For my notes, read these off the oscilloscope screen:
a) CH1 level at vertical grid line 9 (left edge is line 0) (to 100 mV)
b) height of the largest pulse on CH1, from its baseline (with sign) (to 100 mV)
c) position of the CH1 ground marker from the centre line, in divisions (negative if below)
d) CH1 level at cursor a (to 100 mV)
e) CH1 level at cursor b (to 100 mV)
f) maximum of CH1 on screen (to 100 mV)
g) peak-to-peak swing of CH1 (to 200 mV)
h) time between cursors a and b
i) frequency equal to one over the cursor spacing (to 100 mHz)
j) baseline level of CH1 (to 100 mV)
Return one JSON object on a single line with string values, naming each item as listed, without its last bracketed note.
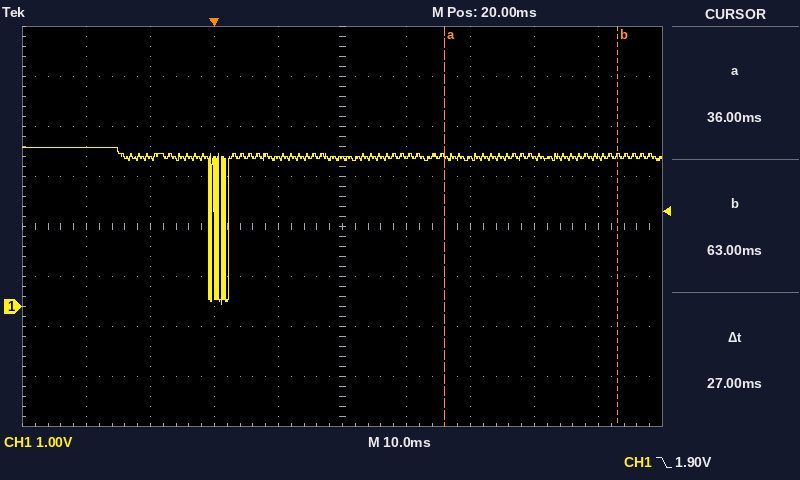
{"CH1 level at vertical grid line 9 (left edge is line 0)": "3.0 V", "height of the largest pulse on CH1, from its baseline (with sign)": "-2.9 V", "position of the CH1 ground marker from the centre line, in divisions": "-1.6 div", "CH1 level at cursor a": "3.0 V", "CH1 level at cursor b": "3.0 V", "maximum of CH1 on screen": "3.2 V", "peak-to-peak swing of CH1": "3.2 V", "time between cursors a and b": "27 ms", "frequency equal to one over the cursor spacing": "37.0 Hz", "baseline level of CH1": "3.0 V"}
